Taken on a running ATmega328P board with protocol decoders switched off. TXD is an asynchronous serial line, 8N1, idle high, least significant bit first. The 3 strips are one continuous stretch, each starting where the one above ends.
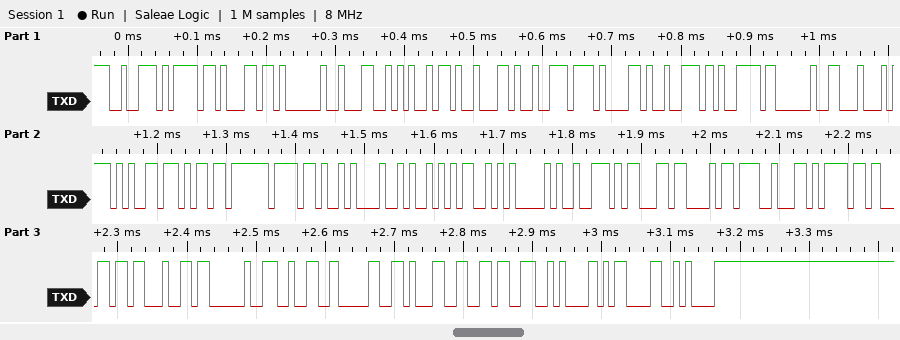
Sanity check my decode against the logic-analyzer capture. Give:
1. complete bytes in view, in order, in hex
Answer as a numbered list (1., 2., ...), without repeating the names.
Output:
1. 72 6F 6C 20 4C 69 62 72 61 72 79 20 44 65 6D 6F 0A 4A 4D 41 72 63 68 62 6F 6C 64 20 32 30 31 36 0A 0D 0A
